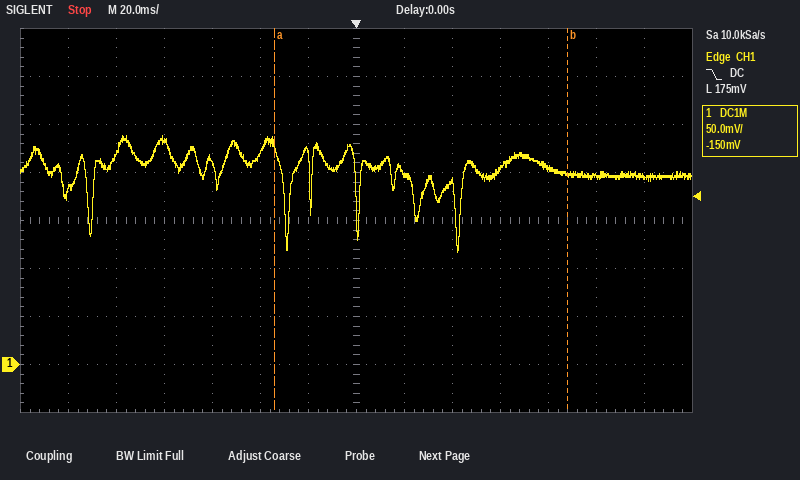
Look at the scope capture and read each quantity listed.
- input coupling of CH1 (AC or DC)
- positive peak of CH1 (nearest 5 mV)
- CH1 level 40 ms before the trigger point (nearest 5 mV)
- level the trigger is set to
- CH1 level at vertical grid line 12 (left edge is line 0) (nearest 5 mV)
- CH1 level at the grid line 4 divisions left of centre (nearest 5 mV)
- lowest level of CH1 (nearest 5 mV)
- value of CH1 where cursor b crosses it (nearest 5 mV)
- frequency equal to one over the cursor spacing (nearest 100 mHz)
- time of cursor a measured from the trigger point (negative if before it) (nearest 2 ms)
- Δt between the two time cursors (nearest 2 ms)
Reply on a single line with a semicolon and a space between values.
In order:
DC; 240 mV; 220 mV; 175 mV; 195 mV; 235 mV; 115 mV; 200 mV; 8.2 Hz; -34 ms; 122 ms
